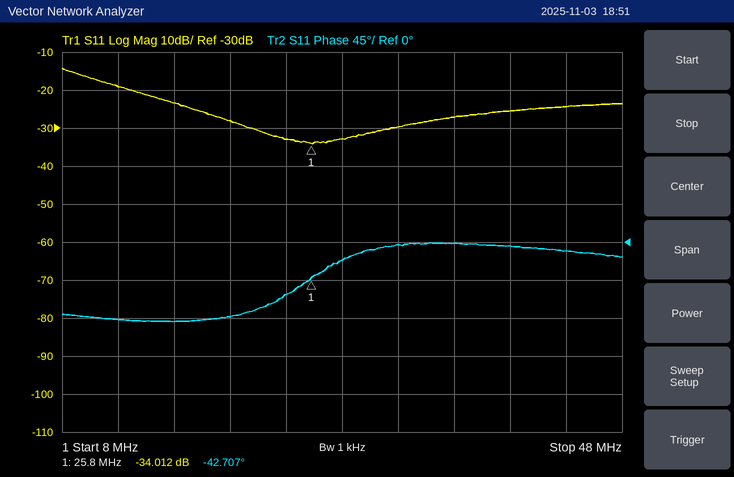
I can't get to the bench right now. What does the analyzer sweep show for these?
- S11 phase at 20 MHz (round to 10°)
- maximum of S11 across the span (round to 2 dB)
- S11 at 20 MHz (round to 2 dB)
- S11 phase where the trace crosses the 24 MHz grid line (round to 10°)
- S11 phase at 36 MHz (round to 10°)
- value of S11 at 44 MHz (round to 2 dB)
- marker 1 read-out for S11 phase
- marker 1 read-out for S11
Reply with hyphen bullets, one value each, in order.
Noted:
- -90°
- -14 dB
- -28 dB
- -60°
- 0°
- -24 dB
- -42.707°
- -34.012 dB
